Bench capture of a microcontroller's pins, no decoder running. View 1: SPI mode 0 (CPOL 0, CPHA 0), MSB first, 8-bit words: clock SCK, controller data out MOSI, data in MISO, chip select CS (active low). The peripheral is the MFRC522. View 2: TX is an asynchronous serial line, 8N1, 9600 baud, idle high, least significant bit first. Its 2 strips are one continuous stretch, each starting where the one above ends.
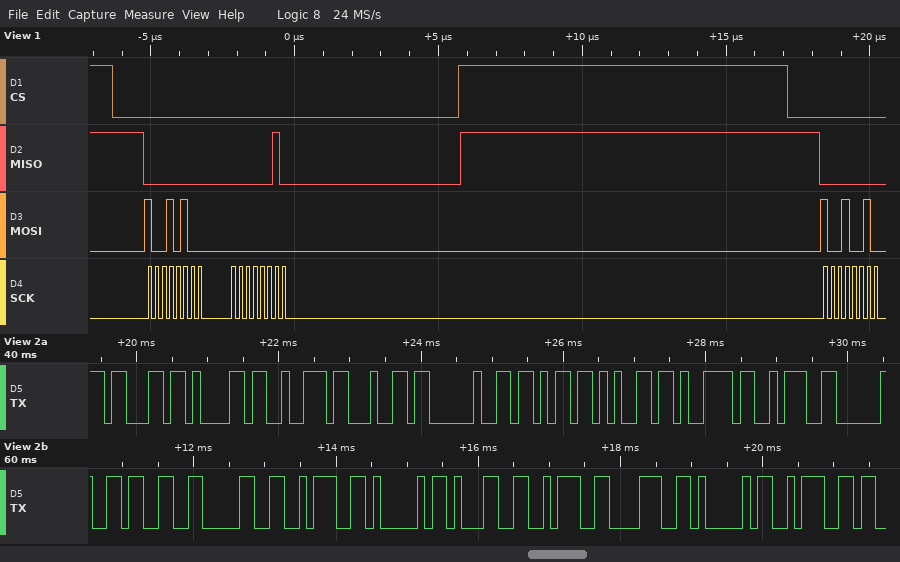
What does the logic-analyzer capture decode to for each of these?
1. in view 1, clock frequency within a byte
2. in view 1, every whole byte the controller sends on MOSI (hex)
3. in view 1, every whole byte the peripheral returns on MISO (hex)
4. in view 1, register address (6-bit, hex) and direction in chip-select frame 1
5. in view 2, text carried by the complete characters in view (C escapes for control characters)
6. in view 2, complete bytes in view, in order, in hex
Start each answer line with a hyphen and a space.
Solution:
- 4 MHz
- 94 00 92
- 00 02 00
- 0x0A read
- "card key: 30:A1:8A:"
- 63 61 72 64 20 6B 65 79 3A 20 33 30 3A 41 31 3A 38 41 3A
